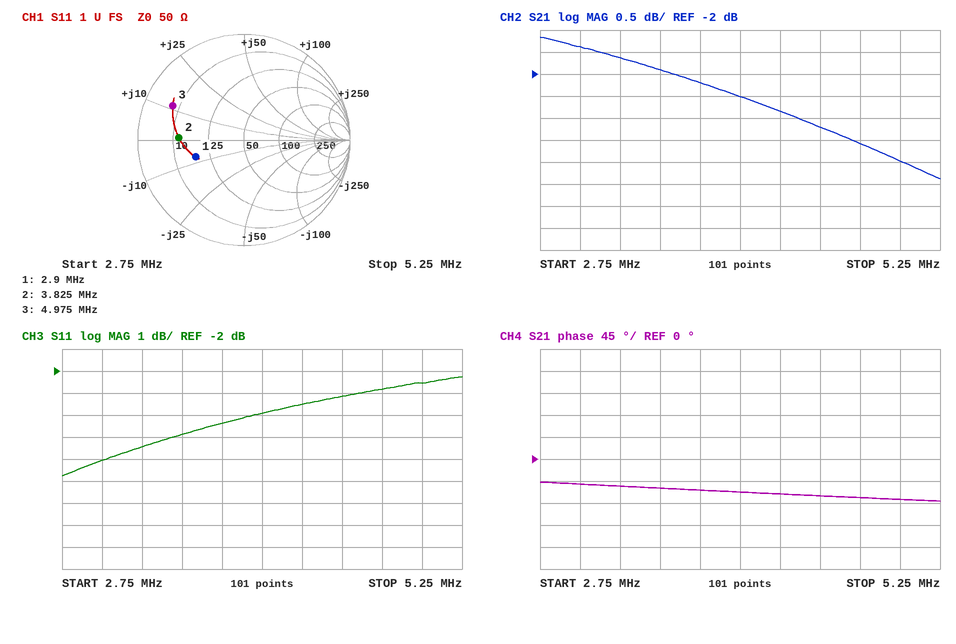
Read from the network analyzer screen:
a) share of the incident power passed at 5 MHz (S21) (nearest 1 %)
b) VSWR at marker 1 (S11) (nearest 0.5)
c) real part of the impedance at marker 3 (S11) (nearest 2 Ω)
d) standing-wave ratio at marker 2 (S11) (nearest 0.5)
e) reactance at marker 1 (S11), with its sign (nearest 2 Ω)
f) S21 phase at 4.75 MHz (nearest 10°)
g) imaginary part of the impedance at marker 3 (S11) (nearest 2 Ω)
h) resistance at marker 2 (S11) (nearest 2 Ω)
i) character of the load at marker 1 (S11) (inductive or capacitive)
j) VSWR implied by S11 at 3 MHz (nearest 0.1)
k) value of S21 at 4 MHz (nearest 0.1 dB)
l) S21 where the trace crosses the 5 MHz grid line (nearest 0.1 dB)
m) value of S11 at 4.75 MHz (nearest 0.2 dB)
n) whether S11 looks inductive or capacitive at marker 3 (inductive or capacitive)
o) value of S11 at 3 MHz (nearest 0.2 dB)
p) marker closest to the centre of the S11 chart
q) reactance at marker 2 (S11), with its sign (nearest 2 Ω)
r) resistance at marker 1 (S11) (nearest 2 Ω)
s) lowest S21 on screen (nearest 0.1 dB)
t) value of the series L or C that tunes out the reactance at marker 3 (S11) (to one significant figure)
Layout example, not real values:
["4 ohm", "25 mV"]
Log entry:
["40 %", "3.0", "8 Ω", "4.0", "-8 Ω", "-80°", "+12 Ω", "12 Ω", "capacitive", "3.0", "-2.5 dB", "-4.0 dB", "-2.8 dB", "inductive", "-6.0 dB", "marker 1", "0 Ω", "18 Ω", "-4.4 dB", "3 nF"]
